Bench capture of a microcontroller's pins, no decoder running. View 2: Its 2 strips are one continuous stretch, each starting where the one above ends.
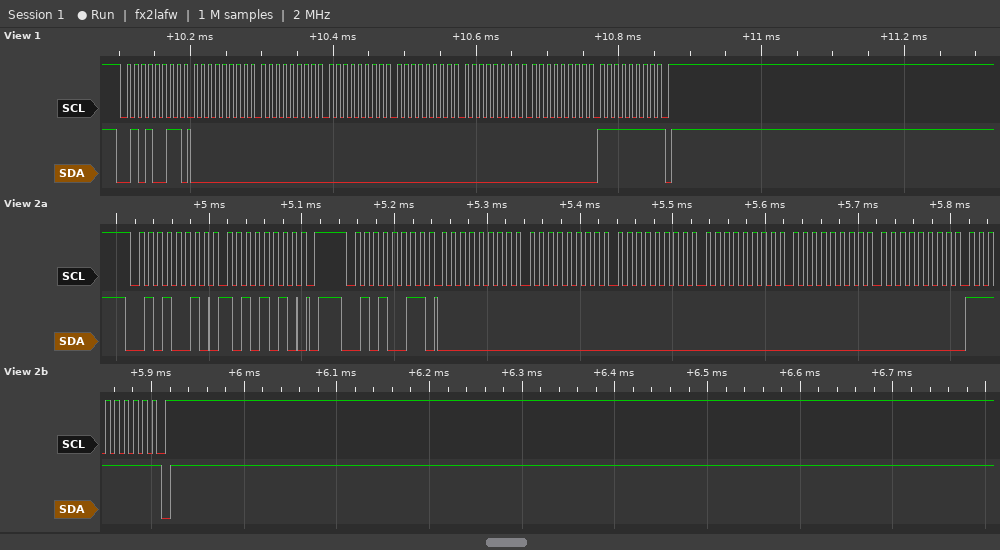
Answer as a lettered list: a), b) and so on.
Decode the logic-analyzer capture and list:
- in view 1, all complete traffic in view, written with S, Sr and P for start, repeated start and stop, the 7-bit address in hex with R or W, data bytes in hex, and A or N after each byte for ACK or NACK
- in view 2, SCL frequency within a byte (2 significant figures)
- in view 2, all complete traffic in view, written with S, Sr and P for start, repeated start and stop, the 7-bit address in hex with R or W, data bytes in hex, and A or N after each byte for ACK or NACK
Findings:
a) S 29R A 00 A 00 A 00 A 00 A 00 A 00 A FF N P
b) 100 kHz
c) S 29W A AA A P S 29R A 00 A 00 A 00 A 00 A 00 A 00 A FF N P
